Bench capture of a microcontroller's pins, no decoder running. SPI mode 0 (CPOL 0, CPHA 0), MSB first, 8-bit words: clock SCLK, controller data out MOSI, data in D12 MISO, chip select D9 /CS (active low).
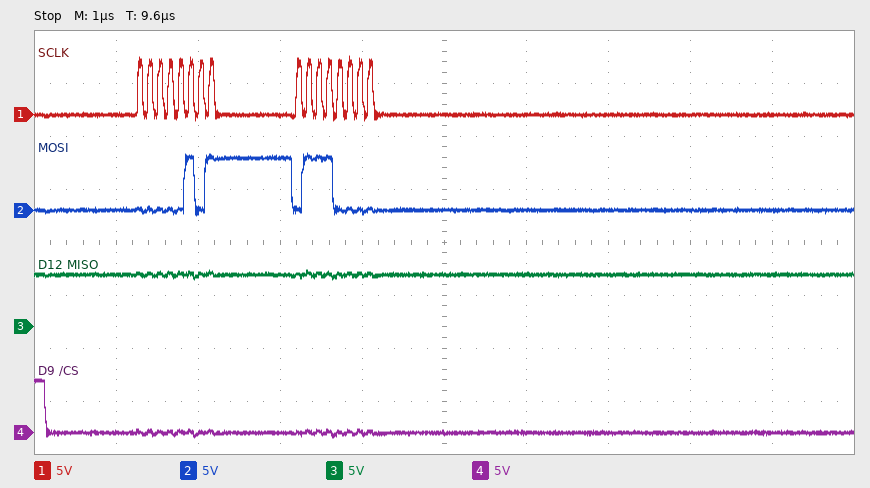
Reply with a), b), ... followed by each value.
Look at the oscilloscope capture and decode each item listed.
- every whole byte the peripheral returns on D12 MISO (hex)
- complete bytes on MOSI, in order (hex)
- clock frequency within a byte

a) FF FF
b) 05 70
c) 8 MHz
